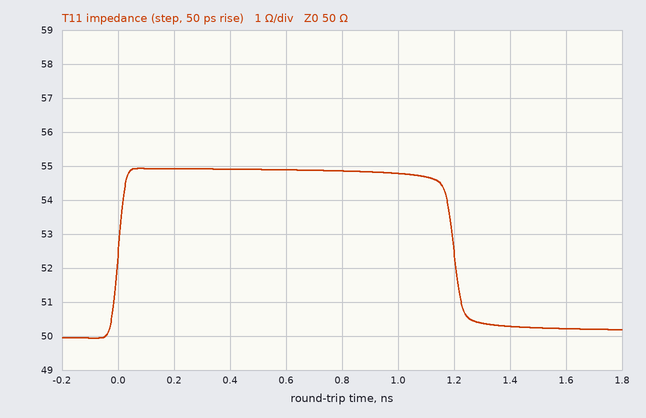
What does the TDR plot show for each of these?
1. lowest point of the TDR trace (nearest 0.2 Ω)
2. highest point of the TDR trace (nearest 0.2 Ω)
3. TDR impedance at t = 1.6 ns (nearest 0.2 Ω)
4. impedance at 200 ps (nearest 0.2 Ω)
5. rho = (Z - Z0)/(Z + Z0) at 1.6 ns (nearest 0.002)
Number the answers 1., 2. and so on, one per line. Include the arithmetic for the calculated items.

1. 50.0 Ω
2. 55.0 Ω
3. 50.2 Ω
4. 55.0 Ω
5. (50.2 − 50)/(50.2 + 50) ≈ +0.002
